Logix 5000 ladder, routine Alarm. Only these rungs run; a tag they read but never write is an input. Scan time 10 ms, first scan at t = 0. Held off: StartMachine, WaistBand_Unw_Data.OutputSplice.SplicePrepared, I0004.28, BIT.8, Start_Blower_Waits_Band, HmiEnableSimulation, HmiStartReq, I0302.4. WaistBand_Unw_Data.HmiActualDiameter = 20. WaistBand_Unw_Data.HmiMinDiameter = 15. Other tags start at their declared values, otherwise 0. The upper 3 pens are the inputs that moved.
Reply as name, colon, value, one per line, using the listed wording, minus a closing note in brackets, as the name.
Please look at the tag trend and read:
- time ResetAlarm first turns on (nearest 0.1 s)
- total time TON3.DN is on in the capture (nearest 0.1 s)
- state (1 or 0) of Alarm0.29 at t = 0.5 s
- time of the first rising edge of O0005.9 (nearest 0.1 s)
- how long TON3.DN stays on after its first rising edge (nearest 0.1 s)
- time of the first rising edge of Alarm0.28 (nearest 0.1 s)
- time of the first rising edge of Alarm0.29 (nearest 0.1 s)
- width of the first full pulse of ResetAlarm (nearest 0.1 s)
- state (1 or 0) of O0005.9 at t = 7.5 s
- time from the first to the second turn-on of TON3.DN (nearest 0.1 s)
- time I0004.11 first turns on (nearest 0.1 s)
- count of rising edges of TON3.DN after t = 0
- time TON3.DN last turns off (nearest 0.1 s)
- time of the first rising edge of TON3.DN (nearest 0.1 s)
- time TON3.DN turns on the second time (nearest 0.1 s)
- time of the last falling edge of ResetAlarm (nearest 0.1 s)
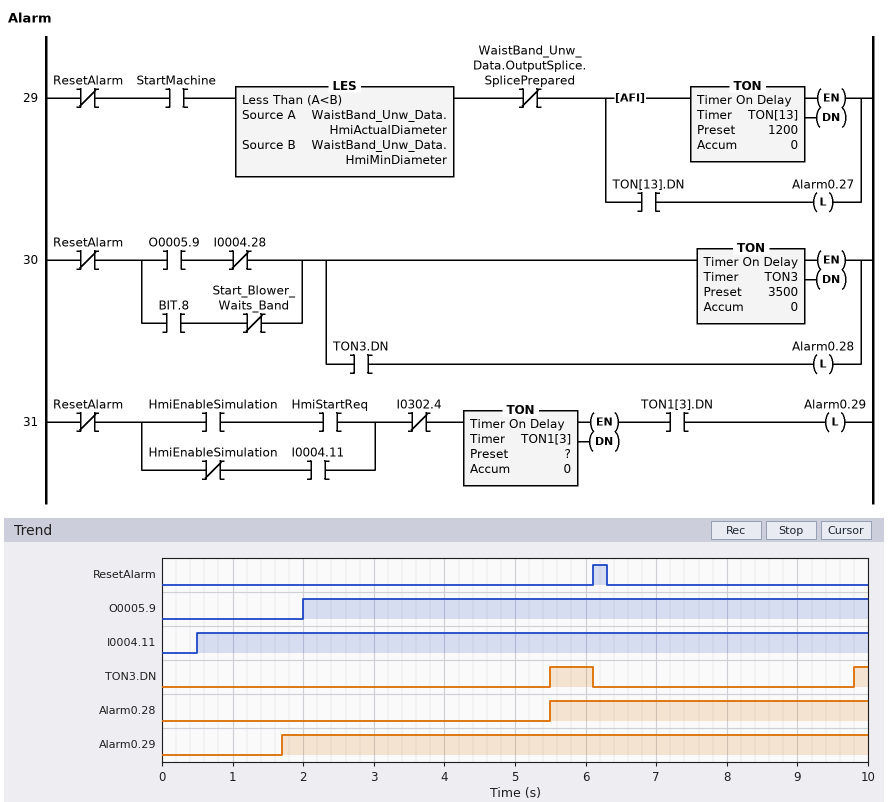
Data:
time ResetAlarm first turns on: 6.1 s
total time TON3.DN is on in the capture: 0.8 s
state (1 or 0) of Alarm0.29 at t = 0.5 s: 0
time of the first rising edge of O0005.9: 2.0 s
how long TON3.DN stays on after its first rising edge: 0.6 s
time of the first rising edge of Alarm0.28: 5.5 s
time of the first rising edge of Alarm0.29: 1.7 s
width of the first full pulse of ResetAlarm: 0.2 s
state (1 or 0) of O0005.9 at t = 7.5 s: 1
time from the first to the second turn-on of TON3.DN: 4.3 s
time I0004.11 first turns on: 0.5 s
count of rising edges of TON3.DN after t = 0: 2
time TON3.DN last turns off: 6.1 s
time of the first rising edge of TON3.DN: 5.5 s
time TON3.DN turns on the second time: 9.8 s
time of the last falling edge of ResetAlarm: 6.3 s
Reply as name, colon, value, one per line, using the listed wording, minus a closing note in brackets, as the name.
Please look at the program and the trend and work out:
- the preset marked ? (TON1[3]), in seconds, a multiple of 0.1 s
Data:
the preset marked ? (TON1[3]), in seconds, a multiple of 0.1 s: 1.2 s
